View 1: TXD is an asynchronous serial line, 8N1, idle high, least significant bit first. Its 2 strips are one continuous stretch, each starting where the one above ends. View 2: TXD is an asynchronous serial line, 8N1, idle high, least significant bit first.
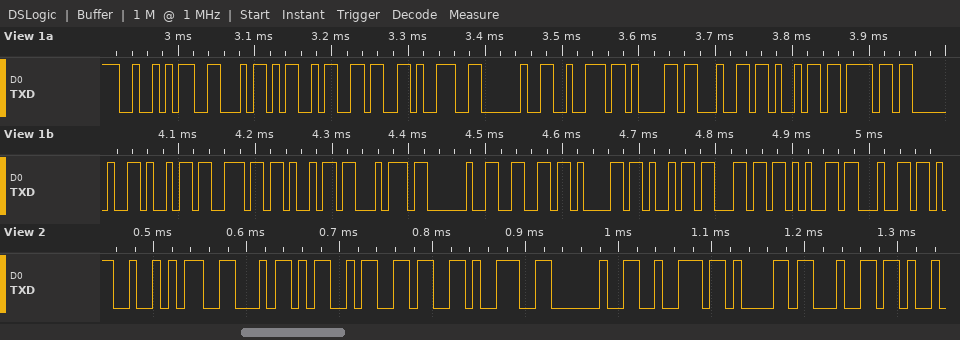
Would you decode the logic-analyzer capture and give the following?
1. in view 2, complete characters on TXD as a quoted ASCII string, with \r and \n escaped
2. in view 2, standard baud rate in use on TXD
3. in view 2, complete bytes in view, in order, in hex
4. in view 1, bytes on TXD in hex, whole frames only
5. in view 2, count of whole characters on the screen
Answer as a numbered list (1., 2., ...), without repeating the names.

1. "RFM69 rad"
2. 115200 baud
3. 52 46 4D 36 39 20 72 61 64
4. 52 46 4D 36 39 20 72 61 64 69 6F 20 69 6E 69 74 20 66 61 69 6C 65 64
5. 9
